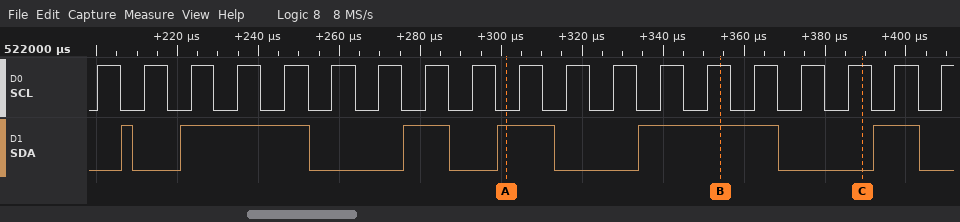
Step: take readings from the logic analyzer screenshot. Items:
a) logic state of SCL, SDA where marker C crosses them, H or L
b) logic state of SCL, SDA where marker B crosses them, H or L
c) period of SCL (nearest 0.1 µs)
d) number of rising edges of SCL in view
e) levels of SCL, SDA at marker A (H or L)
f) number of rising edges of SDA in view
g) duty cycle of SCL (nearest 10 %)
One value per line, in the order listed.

SCL=H, SDA=L
SCL=H, SDA=H
11.6 µs
19
SCL=L, SDA=H
6
50 %
